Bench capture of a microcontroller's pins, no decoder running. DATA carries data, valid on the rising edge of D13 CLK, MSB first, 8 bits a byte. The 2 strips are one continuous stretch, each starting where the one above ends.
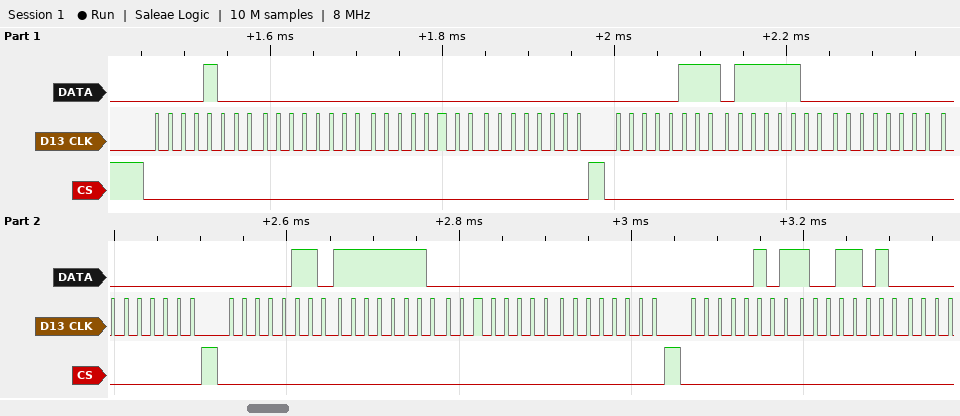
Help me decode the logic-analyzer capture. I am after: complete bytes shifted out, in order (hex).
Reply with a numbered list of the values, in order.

1. 08 00 00 00 07 7C 00 00 06 FE 00 00 05 9A
